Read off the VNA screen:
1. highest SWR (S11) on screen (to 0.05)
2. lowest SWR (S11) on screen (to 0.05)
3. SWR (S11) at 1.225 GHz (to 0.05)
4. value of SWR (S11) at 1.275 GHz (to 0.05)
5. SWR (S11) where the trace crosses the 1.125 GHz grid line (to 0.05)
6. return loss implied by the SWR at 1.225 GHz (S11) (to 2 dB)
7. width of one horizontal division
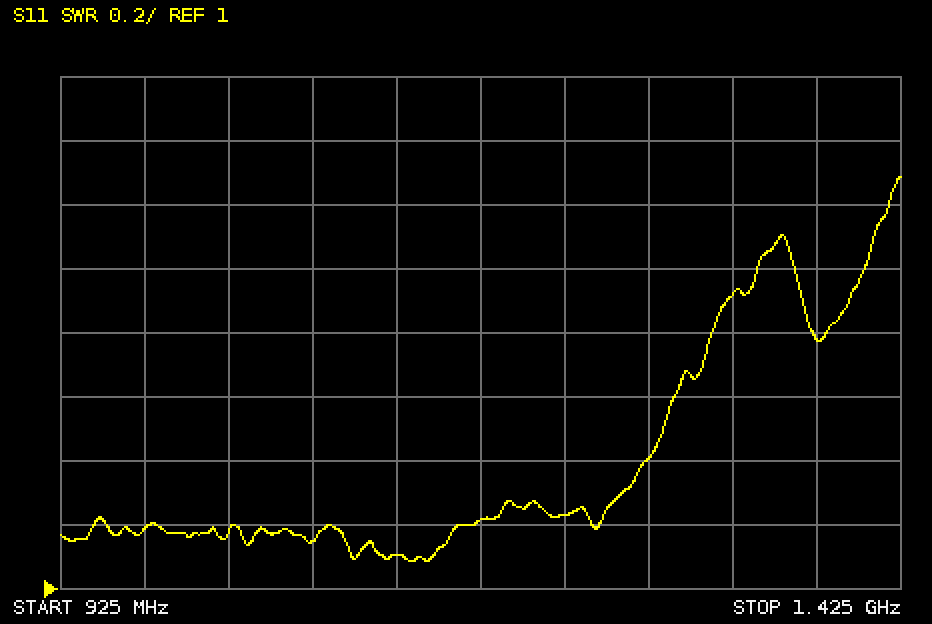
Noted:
2.30
1.10
1.25
1.40
1.10
20 dB
50 MHz
